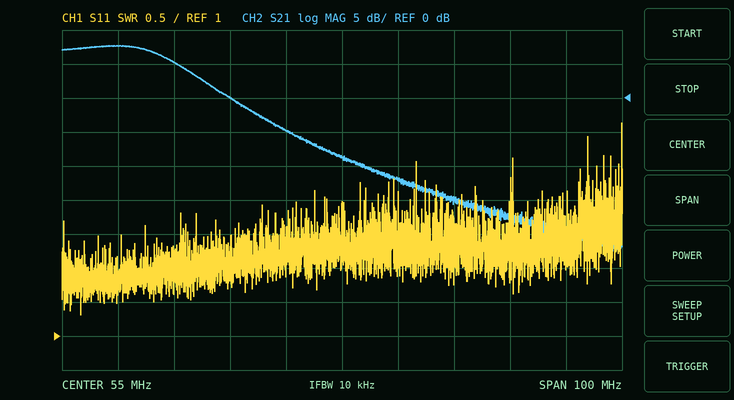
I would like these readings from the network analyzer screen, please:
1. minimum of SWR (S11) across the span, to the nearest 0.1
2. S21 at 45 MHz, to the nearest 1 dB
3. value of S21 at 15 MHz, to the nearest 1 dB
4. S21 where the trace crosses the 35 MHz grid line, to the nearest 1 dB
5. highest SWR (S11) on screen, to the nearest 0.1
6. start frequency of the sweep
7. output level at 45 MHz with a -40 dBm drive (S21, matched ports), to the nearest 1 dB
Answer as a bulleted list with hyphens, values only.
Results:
- 1.3
- -5 dB
- 8 dB
- 0 dB
- 4.1
- 5 MHz
- -45 dBm
